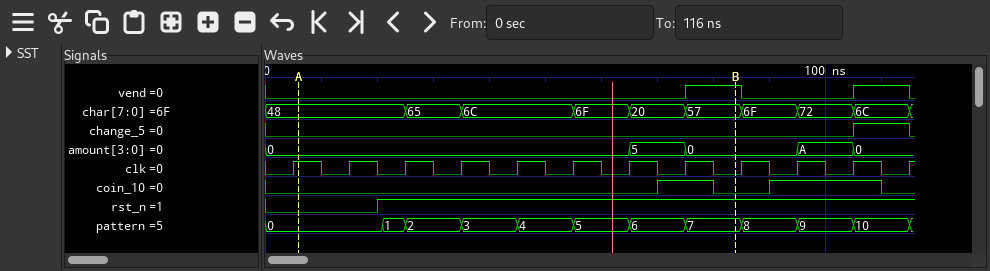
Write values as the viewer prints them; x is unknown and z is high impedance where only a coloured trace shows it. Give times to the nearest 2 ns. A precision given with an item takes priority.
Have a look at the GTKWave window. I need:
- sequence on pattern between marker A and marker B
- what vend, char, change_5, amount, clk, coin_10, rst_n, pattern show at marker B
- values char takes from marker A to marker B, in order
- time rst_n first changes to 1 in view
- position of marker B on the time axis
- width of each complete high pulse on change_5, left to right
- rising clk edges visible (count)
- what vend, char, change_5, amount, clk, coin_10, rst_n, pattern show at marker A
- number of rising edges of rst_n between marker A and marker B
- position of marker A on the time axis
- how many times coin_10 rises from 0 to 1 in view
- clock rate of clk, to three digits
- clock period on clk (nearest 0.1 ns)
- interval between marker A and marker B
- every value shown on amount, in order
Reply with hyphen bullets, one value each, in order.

- 0, 1, 2, 3, 4, 5, 6, 7
- vend=1, char=57, change_5=0, amount=0, clk=0, coin_10=0, rst_n=1, pattern=7
- 48, 65, 6C, 6F, 20, 57
- 20 ns
- 84 ns
- 10 ns
- 12
- vend=0, char=48, change_5=0, amount=0, clk=1, coin_10=0, rst_n=0, pattern=0
- 1
- 6 ns
- 2
- 100 MHz
- 10 ns
- 78 ns
- 0, 5, 0, A, 0
